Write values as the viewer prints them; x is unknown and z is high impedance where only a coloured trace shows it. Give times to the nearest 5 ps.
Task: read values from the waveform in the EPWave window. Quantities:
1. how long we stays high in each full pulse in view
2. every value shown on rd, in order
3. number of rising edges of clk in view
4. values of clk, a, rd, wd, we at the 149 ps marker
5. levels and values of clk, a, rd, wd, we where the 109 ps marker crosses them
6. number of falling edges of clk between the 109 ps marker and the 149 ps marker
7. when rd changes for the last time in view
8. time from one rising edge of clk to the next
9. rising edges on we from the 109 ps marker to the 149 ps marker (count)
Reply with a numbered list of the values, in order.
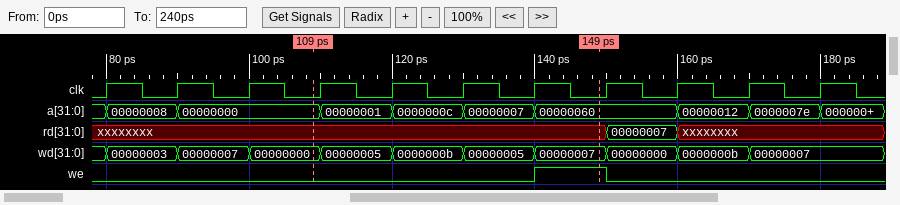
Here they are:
1. 10 ps
2. xxxxxxxx, 00000007, xxxxxxxx
3. 11
4. clk=0, a=00000060, rd=xxxxxxxx, wd=00000007, we=1
5. clk=0, a=00000000, rd=xxxxxxxx, wd=00000000, we=0
6. 4
7. 160 ps
8. 10 ps
9. 1
